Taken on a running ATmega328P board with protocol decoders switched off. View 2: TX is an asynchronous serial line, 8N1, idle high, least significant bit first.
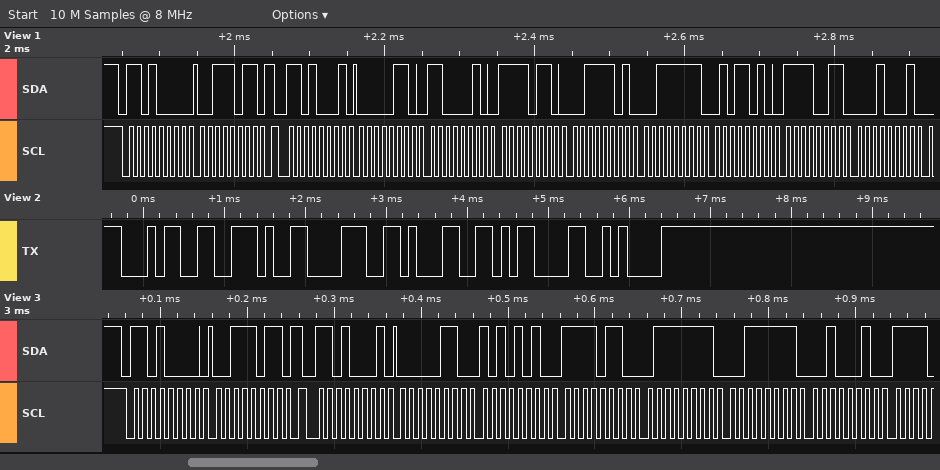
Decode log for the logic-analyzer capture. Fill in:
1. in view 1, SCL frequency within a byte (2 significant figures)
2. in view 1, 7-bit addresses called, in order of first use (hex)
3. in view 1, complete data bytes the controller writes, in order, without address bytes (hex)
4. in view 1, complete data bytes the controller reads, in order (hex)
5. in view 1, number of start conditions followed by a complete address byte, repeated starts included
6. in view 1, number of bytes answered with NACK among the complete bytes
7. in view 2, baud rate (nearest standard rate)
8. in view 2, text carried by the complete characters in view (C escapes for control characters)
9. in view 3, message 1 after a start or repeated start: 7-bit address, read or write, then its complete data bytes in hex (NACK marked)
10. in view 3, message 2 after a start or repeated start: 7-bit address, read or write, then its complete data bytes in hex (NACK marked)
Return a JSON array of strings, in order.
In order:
["100 kHz", "0x68", "3B", "06 C2 F6 3D 3F 5A F3 11", "2", "0", "9600 baud", "\"4.81\\r\\n\"", "0x68 write: 3B", "0x68 read: 06 AA F6 7F 3F 22"]
